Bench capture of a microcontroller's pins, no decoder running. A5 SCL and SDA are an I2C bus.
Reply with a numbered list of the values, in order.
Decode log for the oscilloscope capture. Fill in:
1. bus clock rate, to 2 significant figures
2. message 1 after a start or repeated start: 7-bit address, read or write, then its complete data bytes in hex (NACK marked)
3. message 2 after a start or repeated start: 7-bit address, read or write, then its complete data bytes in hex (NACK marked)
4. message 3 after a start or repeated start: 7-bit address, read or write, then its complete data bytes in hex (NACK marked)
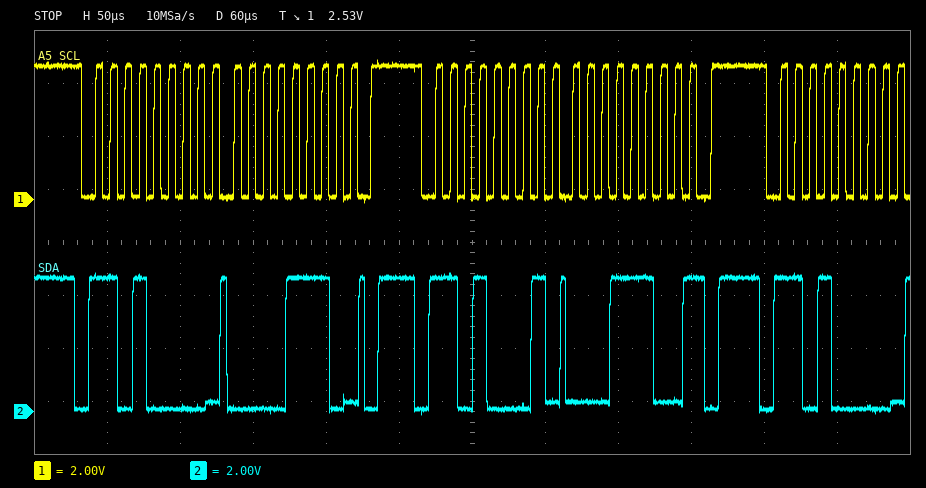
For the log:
1. 100 kHz
2. 0x68 write: 0E
3. 0x68 read: 1C NACK
4. 0x68 write
